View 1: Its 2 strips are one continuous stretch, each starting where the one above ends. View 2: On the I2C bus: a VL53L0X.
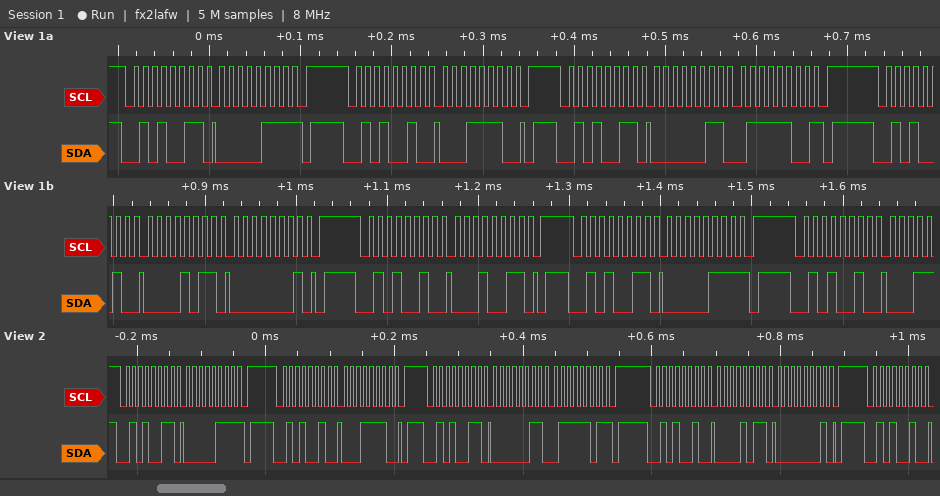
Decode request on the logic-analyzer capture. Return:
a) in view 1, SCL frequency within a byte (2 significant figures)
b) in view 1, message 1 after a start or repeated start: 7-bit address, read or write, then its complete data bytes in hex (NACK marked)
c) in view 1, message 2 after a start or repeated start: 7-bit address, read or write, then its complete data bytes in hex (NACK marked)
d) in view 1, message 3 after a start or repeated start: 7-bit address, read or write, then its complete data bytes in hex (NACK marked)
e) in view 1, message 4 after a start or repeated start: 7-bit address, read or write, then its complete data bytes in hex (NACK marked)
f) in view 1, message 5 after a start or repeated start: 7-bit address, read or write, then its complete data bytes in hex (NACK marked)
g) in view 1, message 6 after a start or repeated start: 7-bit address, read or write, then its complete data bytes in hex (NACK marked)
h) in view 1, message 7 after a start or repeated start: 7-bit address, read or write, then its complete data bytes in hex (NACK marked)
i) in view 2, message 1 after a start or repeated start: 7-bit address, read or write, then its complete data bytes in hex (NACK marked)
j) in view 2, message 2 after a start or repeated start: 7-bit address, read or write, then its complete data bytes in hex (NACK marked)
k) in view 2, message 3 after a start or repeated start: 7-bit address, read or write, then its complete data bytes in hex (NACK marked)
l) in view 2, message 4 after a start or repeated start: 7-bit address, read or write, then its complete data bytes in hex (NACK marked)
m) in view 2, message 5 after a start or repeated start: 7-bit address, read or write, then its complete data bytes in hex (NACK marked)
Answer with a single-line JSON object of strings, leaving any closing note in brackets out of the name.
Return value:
{"in view 1, SCL frequency within a byte": "100 kHz", "in view 1, message 1 after a start or repeated start: 7-bit address, read or write, then its complete data bytes in hex": "0x29 read: 07 NACK", "in view 1, message 2 after a start or repeated start: 7-bit address, read or write, then its complete data bytes in hex": "0x29 write: 1E", "in view 1, message 3 after a start or repeated start: 7-bit address, read or write, then its complete data bytes in hex": "0x29 read: 03 7C NACK", "in view 1, message 4 after a start or repeated start: 7-bit address, read or write, then its complete data bytes in hex": "0x29 write: 0B 01", "in view 1, message 5 after a start or repeated start: 7-bit address, read or write, then its complete data bytes in hex": "0x29 write: 13", "in view 1, message 6 after a start or repeated start: 7-bit address, read or write, then its complete data bytes in hex": "0x29 read: 07 NACK", "in view 1, message 7 after a start or repeated start: 7-bit address, read or write, then its complete data bytes in hex": "0x29 write", "in view 2, message 1 after a start or repeated start: 7-bit address, read or write, then its complete data bytes in hex": "0x29 read: 07 NACK", "in view 2, message 2 after a start or repeated start: 7-bit address, read or write, then its complete data bytes in hex": "0x29 write: 1E", "in view 2, message 3 after a start or repeated start: 7-bit address, read or write, then its complete data bytes in hex": "0x29 read: 03 7D NACK", "in view 2, message 4 after a start or repeated start: 7-bit address, read or write, then its complete data bytes in hex": "0x29 write: 0B 01", "in view 2, message 5 after a start or repeated start: 7-bit address, read or write, then its complete data bytes in hex": "0x29 write"}
